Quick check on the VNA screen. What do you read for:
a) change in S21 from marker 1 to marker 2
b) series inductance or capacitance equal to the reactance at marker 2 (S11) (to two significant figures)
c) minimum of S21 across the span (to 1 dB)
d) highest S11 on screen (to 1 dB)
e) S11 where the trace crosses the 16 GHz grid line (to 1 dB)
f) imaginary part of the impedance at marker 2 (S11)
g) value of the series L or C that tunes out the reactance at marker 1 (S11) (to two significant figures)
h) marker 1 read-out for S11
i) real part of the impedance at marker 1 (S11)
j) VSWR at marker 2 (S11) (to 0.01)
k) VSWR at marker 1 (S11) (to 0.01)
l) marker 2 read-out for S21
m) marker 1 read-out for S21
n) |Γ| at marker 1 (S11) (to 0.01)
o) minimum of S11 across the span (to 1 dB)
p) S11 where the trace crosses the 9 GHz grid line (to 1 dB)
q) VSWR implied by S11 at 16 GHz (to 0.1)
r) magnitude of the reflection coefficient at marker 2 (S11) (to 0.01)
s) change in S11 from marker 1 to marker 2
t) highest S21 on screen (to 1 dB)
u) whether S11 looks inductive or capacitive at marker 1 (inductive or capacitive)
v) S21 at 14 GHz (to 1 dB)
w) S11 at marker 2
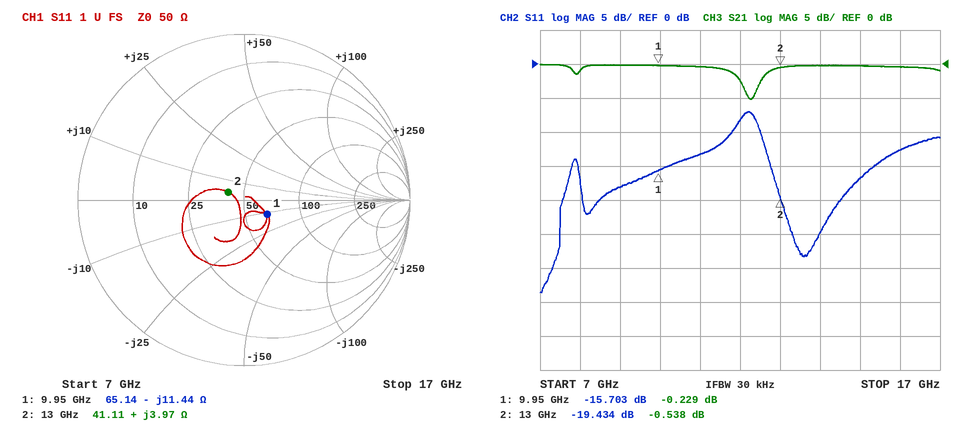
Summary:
-0.309 dB
49 pH
-5 dB
-7 dB
-13 dB
+3.97 Ω
180 pH
-15.703 dB
65.14 Ω
1.24
1.39
-0.538 dB
-0.229 dB
0.16
-34 dB
-18 dB
1.6
0.11
-3.731 dB
0 dB
capacitive
0 dB
-19.434 dB
